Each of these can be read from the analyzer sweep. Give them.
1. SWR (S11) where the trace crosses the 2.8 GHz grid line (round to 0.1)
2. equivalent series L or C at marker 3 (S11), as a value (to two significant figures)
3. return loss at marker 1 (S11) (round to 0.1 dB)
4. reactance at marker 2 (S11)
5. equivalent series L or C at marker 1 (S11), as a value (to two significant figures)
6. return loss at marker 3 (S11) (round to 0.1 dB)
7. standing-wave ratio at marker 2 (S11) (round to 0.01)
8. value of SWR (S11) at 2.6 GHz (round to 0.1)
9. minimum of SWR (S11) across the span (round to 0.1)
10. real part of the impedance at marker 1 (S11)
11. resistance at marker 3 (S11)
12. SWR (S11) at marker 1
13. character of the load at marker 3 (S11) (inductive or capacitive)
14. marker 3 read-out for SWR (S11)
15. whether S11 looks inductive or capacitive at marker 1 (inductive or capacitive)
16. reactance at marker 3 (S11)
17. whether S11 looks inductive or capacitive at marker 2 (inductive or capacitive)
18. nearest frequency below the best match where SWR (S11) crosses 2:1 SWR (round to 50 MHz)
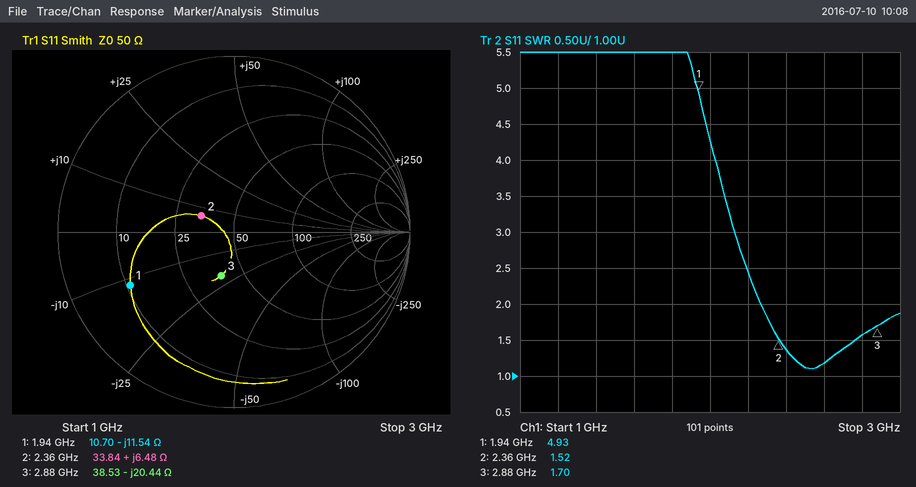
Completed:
1.6
2.7 pF
3.6 dB
+6.48 Ω
7.1 pF
11.8 dB
1.52
1.2
1.1
10.70 Ω
38.53 Ω
4.93
capacitive
1.70
capacitive
-20.44 Ω
inductive
2.25 GHz
